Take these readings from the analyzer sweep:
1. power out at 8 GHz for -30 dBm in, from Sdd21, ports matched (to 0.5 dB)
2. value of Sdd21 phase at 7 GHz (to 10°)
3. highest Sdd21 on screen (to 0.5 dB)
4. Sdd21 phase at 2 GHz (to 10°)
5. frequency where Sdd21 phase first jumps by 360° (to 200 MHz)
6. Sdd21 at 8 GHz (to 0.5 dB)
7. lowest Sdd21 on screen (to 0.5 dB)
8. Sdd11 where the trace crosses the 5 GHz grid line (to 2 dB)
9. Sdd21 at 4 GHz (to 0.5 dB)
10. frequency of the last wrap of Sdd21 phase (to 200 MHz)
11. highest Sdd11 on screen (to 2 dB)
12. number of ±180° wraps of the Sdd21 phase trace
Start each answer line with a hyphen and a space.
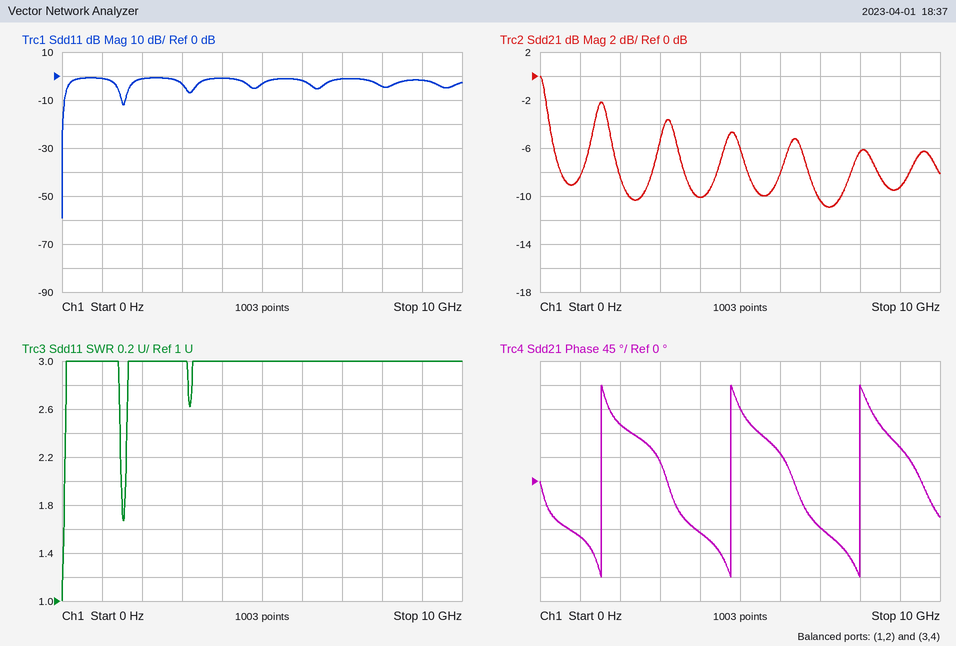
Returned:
- -36.5 dBm
- -90°
- 0.0 dB
- 110°
- 1.6 GHz
- -6.5 dB
- -11.0 dB
- -4 dB
- -10.0 dB
- 8.0 GHz
- 0 dB
- 3
